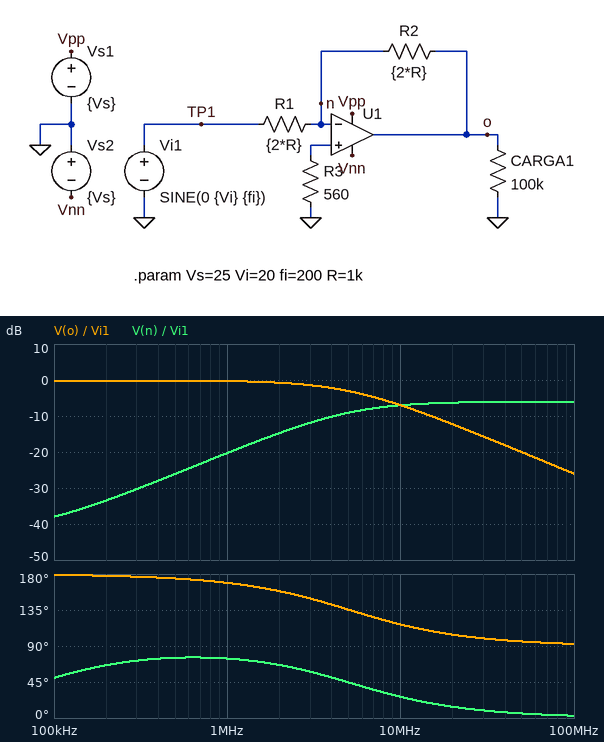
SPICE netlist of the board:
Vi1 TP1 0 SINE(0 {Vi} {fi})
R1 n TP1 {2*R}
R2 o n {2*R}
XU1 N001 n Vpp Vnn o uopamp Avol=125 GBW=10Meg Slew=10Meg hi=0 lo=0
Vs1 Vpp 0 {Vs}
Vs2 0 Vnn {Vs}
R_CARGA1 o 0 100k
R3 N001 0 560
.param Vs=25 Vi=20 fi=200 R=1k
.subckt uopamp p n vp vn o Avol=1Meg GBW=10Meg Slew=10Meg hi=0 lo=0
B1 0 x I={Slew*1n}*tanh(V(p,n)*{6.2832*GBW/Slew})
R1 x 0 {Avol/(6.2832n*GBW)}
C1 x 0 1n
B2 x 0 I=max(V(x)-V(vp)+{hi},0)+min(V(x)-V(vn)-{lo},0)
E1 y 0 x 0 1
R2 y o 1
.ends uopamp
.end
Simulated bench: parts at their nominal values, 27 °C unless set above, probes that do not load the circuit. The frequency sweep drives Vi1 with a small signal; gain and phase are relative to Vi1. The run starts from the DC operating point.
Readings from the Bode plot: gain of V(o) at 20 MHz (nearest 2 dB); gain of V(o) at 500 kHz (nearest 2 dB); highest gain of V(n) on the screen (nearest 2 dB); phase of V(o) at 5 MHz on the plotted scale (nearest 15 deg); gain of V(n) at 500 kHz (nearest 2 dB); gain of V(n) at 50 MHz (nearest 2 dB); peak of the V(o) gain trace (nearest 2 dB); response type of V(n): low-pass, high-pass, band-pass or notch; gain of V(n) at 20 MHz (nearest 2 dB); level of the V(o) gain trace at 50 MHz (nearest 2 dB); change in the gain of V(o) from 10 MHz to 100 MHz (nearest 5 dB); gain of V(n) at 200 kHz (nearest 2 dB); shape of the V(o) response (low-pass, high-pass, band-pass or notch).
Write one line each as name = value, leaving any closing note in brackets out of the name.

gain of V(o) at 20 MHz = -12 dB
gain of V(o) at 500 kHz = 0 dB
highest gain of V(n) on the screen = -6 dB
phase of V(o) at 5 MHz on the plotted scale = 135 deg
gain of V(n) at 500 kHz = -26 dB
gain of V(n) at 50 MHz = -6 dB
peak of the V(o) gain trace = 0 dB
response type of V(n): low-pass, high-pass, band-pass or notch = high-pass
gain of V(n) at 20 MHz = -6 dB
level of the V(o) gain trace at 50 MHz = -20 dB
change in the gain of V(o) from 10 MHz to 100 MHz = -20 dB
gain of V(n) at 200 kHz = -34 dB
shape of the V(o) response = low-pass
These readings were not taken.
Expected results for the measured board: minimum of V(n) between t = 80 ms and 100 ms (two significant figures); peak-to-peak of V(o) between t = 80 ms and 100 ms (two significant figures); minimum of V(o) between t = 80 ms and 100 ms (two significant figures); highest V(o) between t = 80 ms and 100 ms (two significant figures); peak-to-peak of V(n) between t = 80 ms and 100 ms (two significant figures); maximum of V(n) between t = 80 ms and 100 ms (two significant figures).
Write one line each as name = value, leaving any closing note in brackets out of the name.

minimum of V(n) between t = 80 ms and 100 ms = -340 mV
peak-to-peak of V(o) between t = 80 ms and 100 ms = 39 V
minimum of V(o) between t = 80 ms and 100 ms = -19 V
highest V(o) between t = 80 ms and 100 ms = 19 V
peak-to-peak of V(n) between t = 80 ms and 100 ms = 680 mV
maximum of V(n) between t = 80 ms and 100 ms = 340 mV
